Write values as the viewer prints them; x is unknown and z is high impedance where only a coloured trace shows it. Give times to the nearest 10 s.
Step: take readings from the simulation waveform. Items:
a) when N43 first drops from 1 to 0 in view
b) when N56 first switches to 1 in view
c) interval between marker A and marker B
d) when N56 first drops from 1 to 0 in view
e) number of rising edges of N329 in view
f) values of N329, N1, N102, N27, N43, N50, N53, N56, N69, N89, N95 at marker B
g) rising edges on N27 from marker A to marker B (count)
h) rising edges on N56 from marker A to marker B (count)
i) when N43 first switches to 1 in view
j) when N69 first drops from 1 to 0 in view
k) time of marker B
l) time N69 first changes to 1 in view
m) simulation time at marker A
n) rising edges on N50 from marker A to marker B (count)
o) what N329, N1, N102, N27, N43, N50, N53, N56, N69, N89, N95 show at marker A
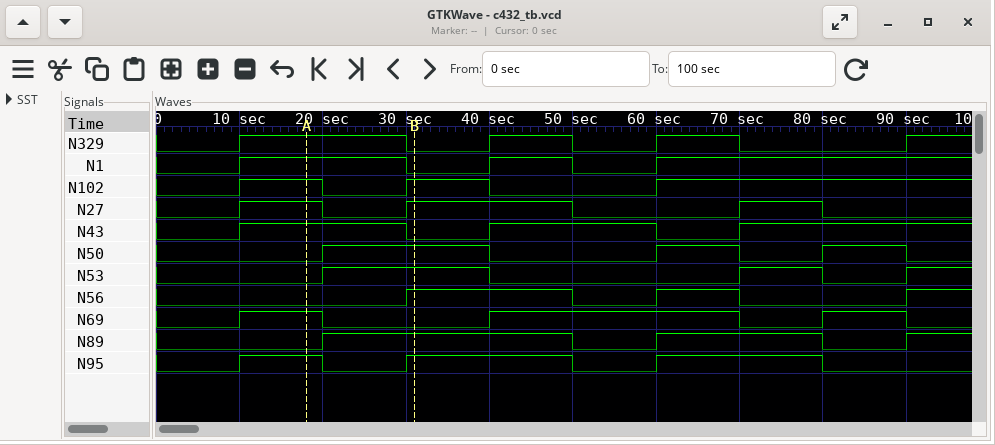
30 s
30 s
10 s
50 s
4
N329=0, N1=0, N102=1, N27=1, N43=0, N50=1, N53=1, N56=1, N69=0, N89=1, N95=1
1
1
10 s
20 s
30 s
10 s
20 s
1
N329=1, N1=1, N102=1, N27=1, N43=1, N50=0, N53=0, N56=0, N69=1, N89=0, N95=1
